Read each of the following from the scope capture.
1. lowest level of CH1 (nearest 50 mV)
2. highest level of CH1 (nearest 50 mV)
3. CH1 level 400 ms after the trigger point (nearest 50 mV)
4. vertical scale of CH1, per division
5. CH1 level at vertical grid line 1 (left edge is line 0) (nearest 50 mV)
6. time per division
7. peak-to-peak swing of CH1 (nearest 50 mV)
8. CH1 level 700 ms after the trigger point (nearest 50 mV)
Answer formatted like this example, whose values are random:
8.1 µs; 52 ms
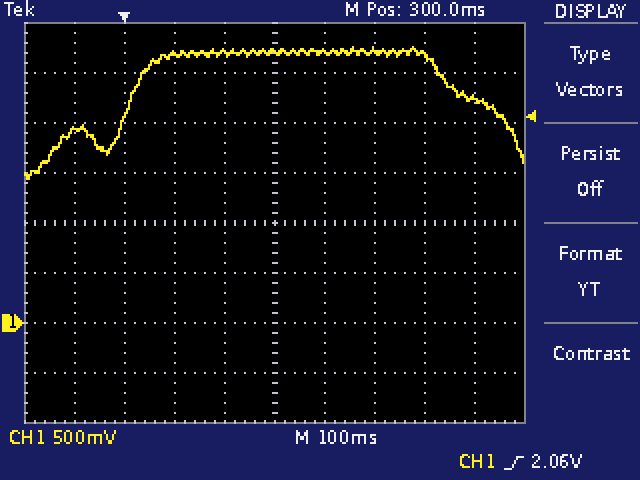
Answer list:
1.45 V; 2.75 V; 2.70 V; 500 mV; 1.95 V; 100 ms; 1.30 V; 2.25 V
